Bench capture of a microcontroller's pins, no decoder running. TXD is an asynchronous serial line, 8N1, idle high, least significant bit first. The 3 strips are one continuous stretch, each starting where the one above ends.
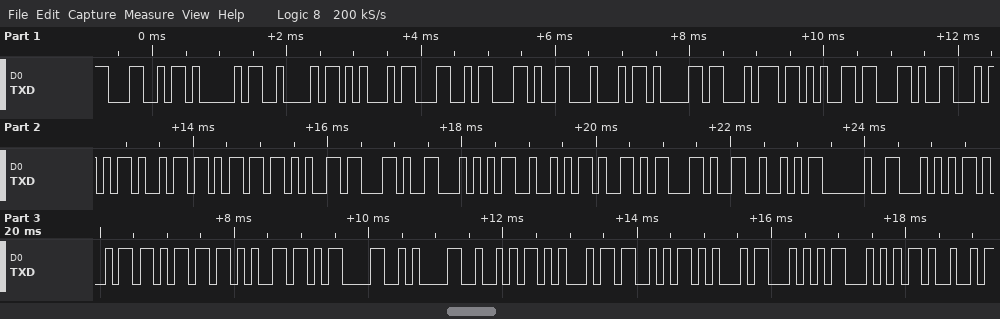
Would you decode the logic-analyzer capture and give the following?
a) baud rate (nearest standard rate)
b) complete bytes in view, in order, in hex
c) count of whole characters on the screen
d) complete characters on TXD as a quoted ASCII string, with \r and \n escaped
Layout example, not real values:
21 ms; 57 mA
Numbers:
9600 baud; 4C 41 42 45 4C 2C 44 61 74 65 2C 54 69 6D 65 2C 54 52 59 2C 52 20 54 69 6D 65 0D 0A 52 45 53 45 54 54 49; 35; "LABEL,Date,Time,TRY,R Time\r\nRESETTI"
